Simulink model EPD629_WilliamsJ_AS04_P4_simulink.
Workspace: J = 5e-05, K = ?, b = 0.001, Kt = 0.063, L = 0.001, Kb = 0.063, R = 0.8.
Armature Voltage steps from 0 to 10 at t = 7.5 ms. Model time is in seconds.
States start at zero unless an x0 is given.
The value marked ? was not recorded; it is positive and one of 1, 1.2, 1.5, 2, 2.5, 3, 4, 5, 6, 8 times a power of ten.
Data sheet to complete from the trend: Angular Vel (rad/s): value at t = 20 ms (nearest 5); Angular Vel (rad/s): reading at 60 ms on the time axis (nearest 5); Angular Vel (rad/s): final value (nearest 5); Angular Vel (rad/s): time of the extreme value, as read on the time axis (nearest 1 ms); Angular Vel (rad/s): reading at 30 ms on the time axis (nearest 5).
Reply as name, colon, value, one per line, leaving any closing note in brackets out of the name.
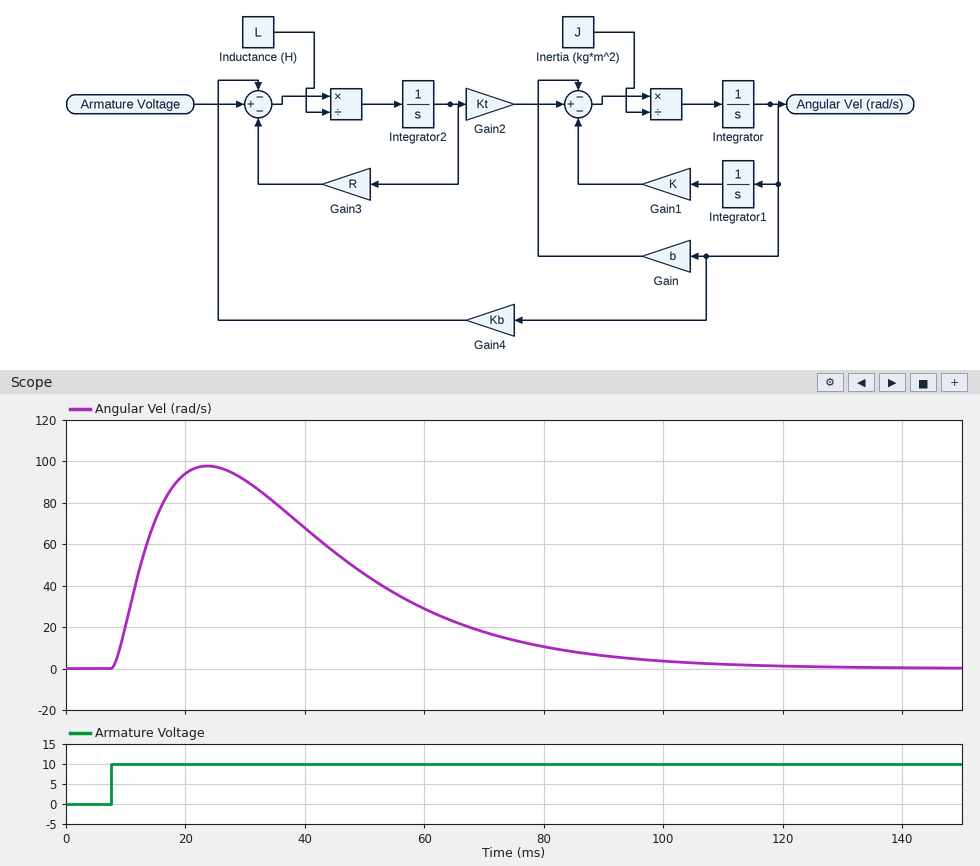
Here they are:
Angular Vel (rad/s): value at t = 20 ms: 95
Angular Vel (rad/s): reading at 60 ms on the time axis: 30
Angular Vel (rad/s): final value: 0
Angular Vel (rad/s): time of the extreme value, as read on the time axis: 24 ms
Angular Vel (rad/s): reading at 30 ms on the time axis: 90
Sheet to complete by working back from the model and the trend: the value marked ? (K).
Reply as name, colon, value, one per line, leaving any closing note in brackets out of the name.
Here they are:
the value marked ?: 0.2
